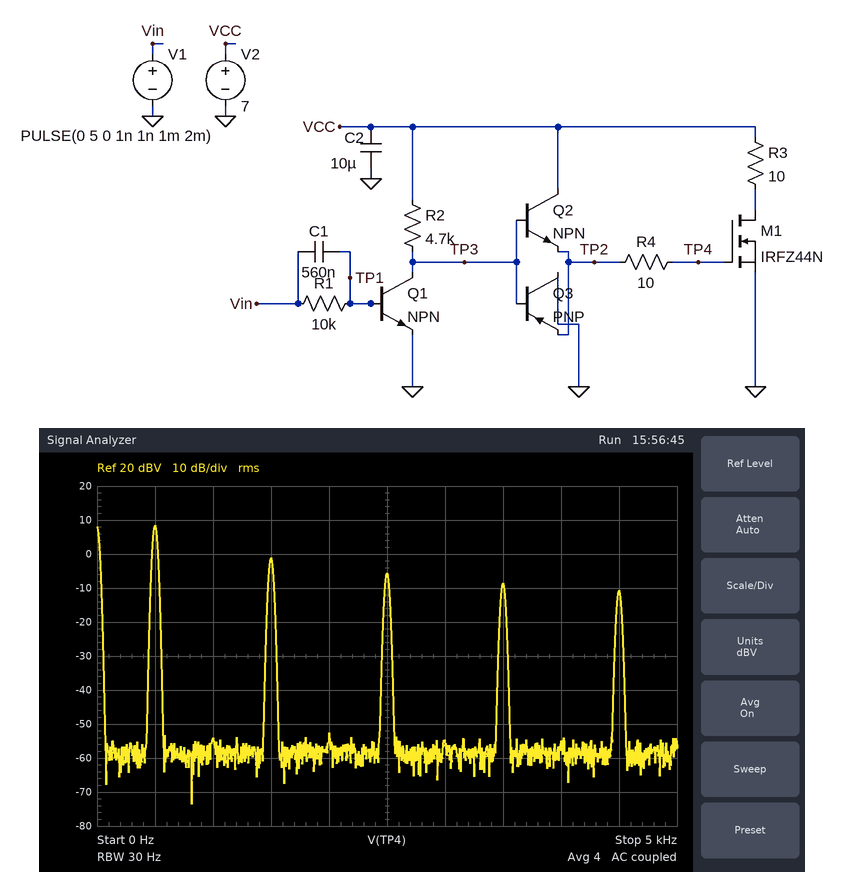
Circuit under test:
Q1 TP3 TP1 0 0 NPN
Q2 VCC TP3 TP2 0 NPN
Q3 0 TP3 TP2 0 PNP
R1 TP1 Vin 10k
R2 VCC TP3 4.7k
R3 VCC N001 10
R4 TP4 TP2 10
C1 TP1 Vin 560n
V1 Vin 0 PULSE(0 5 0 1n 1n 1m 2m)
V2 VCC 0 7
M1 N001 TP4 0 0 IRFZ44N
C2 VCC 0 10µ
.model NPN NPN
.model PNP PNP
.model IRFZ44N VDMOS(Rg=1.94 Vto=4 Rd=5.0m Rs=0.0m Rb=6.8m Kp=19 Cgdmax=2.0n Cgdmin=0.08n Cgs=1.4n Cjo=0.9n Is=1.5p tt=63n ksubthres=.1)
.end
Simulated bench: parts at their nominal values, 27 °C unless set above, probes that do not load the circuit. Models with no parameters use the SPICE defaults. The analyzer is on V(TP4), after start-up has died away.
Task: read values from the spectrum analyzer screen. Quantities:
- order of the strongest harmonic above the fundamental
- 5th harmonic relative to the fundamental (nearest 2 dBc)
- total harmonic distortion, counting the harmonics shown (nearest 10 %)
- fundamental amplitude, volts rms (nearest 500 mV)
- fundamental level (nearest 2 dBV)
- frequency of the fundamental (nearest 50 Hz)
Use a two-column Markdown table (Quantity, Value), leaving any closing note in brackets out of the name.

| Quantity | Value |
|---|---|
| order of the strongest harmonic above the fundamental | 3 |
| 5th harmonic relative to the fundamental | -14 dBc |
| total harmonic distortion, counting the harmonics shown | 40 % |
| fundamental amplitude, volts rms | 2.5 V |
| fundamental level | 8 dBV |
| frequency of the fundamental | 500 Hz |
